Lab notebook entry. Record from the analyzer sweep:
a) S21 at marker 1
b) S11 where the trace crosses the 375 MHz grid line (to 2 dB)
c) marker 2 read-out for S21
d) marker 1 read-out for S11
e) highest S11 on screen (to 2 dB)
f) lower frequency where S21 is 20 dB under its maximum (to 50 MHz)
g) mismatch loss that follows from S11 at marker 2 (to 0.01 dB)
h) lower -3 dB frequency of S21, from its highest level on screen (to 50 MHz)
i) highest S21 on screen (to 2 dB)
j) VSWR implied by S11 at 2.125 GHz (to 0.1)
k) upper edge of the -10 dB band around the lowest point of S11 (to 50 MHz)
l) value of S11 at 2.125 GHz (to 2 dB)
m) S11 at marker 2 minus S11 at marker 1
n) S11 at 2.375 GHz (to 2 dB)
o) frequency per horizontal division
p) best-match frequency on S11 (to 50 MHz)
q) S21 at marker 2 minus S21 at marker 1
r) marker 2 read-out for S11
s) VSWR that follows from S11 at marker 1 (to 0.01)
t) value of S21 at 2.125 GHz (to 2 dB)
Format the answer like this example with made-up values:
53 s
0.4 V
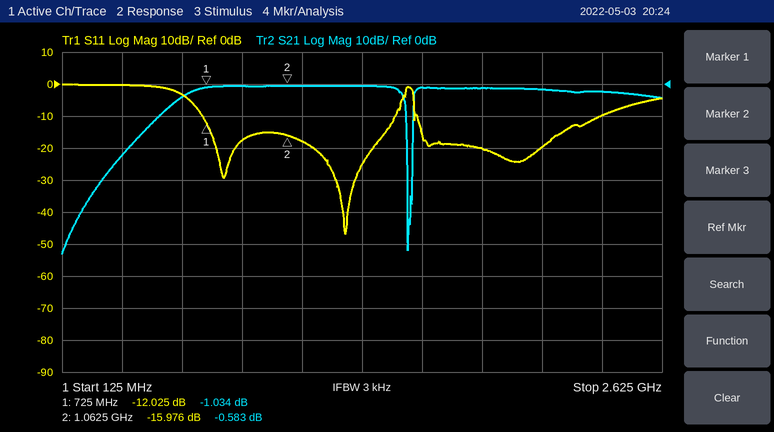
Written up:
-1.034 dB
0 dB
-0.583 dB
-12.025 dB
0 dB
400 MHz
0.11 dB
650 MHz
0 dB
1.2
1.50 GHz
-20 dB
-3.951 dB
-10 dB
250 MHz
1.30 GHz
0.451 dB
-15.976 dB
1.67
-2 dB
